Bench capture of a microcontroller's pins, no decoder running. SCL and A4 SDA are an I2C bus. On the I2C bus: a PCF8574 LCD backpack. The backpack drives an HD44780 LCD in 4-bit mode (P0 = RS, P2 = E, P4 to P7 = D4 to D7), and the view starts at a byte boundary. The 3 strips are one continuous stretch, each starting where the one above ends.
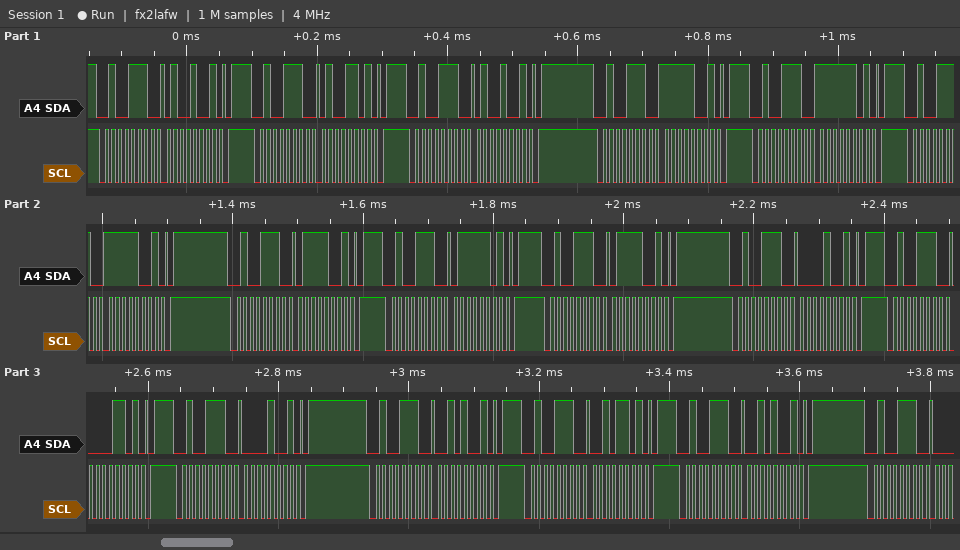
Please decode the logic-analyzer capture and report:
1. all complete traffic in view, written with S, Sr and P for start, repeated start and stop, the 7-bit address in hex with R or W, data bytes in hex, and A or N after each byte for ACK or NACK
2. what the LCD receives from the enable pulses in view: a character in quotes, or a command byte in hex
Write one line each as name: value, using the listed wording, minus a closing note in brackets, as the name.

all complete traffic in view, written with S, Sr and P for start, repeated start and stop, the 7-bit address in hex with R or W, data bytes in hex, and A or N after each byte for ACK or NACK: S 27W A 49 A P S 27W A 4D A P S 27W A 49 A P S 27W A F9 A P S 27W A FD A P S 27W A F9 A P S 27W A 79 A P S 27W A 7D A P S 27W A 79 A P S 27W A 09 A P S 27W A 0D A P S 27W A 09 A P S 27W A 29 A P S 27W A 2D A P S 27W A 29 A P S 27W A
what the LCD receives from the enable pulses in view: a character in quotes, or a command byte in hex: 'O' 'p'
